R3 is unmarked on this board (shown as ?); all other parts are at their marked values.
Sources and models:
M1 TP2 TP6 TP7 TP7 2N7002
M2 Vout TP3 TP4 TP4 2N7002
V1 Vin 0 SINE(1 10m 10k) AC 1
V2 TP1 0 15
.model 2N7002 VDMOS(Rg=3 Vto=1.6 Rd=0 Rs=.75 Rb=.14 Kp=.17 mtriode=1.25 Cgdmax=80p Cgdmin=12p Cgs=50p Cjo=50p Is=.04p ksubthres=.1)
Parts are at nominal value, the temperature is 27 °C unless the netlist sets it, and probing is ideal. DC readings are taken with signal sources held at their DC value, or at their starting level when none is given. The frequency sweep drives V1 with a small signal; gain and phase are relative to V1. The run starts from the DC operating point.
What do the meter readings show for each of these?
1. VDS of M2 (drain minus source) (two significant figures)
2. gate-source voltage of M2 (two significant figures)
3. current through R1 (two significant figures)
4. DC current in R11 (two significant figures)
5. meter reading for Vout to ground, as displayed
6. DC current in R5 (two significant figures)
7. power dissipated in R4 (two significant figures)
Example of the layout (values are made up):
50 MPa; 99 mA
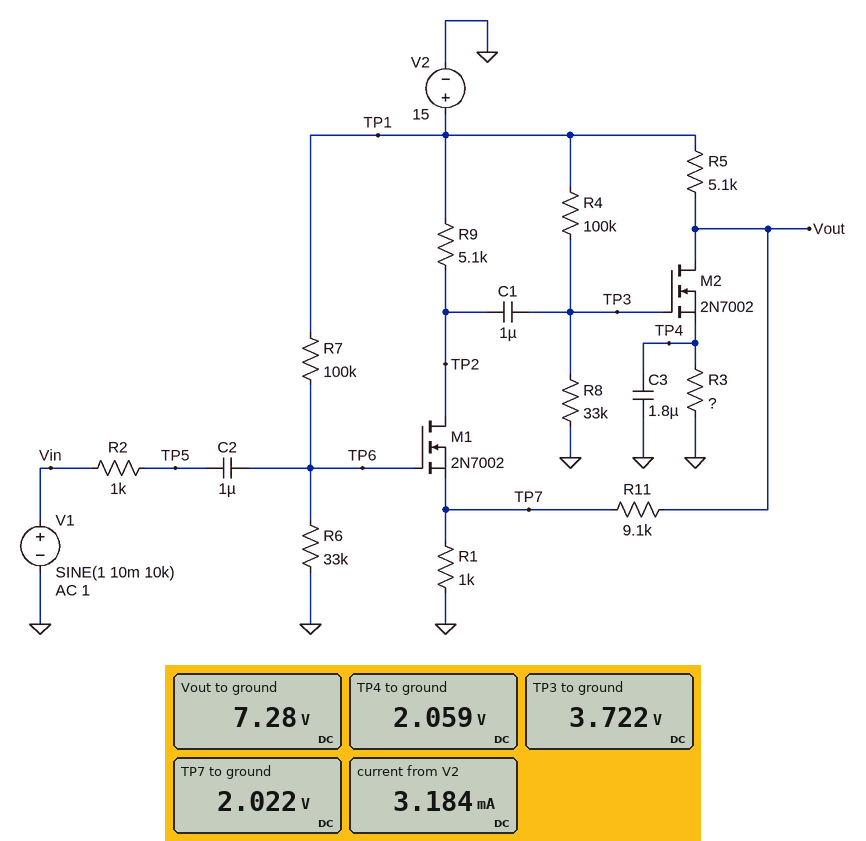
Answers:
5.2 V; 1.7 V; 2.0 mA; 580 µA; 7.28 V; 1.5 mA; 1.3 mW
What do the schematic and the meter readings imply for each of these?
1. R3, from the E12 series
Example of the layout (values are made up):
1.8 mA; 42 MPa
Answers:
2.2 kΩ
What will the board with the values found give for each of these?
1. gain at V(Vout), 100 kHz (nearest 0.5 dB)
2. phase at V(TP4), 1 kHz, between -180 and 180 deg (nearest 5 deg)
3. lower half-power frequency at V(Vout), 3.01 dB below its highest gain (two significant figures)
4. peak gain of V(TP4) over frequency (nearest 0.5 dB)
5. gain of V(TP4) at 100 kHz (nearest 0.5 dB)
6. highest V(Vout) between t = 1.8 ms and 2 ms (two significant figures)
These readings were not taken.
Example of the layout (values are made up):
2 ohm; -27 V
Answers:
19.0 dB; 95 deg; 76 Hz; 7.5 dB; -52.5 dB; 7.4 V
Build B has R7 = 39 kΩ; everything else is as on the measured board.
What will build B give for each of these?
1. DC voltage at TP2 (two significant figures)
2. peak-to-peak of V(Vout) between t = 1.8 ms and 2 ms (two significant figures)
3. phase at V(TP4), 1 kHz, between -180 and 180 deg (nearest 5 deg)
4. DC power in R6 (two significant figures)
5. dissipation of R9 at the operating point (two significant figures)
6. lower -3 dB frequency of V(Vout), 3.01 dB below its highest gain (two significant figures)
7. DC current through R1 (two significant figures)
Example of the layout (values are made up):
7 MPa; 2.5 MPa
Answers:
2.9 V; 1.1 mV; 85 deg; 1.4 mW; 29 mW; 430 kHz; 2.9 mA
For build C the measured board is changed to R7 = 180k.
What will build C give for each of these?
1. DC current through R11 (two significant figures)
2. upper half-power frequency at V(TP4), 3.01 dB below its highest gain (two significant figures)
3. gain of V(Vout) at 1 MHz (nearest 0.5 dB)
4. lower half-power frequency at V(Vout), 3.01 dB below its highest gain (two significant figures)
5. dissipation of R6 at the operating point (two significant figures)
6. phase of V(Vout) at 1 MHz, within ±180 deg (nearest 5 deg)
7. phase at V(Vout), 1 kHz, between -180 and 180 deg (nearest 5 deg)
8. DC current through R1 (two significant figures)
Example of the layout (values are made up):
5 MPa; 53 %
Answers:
660 µA; 130 Hz; 13.5 dB; 100 Hz; 160 µW; -90 deg; 5 deg; 800 µA
